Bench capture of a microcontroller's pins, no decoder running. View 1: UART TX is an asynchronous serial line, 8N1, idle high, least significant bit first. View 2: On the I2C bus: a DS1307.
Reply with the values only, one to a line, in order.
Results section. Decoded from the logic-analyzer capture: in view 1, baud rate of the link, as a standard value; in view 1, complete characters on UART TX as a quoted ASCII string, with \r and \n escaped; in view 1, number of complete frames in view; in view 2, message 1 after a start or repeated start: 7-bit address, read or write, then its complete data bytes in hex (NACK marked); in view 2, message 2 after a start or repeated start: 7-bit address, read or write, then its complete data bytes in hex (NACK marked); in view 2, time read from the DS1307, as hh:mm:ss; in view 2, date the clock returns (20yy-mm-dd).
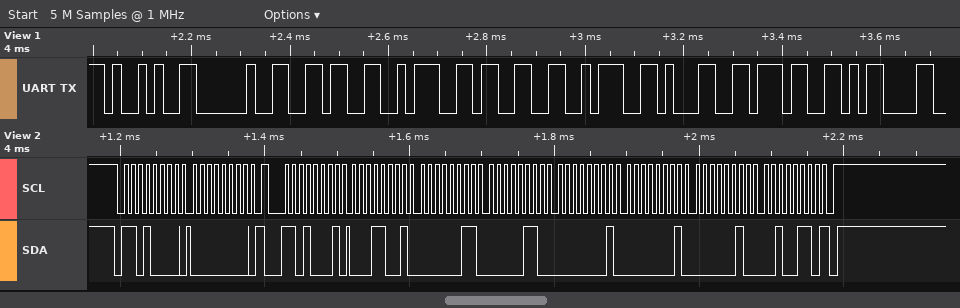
57600 baud
") 6:3:17\r"
9
0x68 write: 00
0x68 read: 19 03 06 01 01 02 26 NACK
06:03:19
2026-02-01
